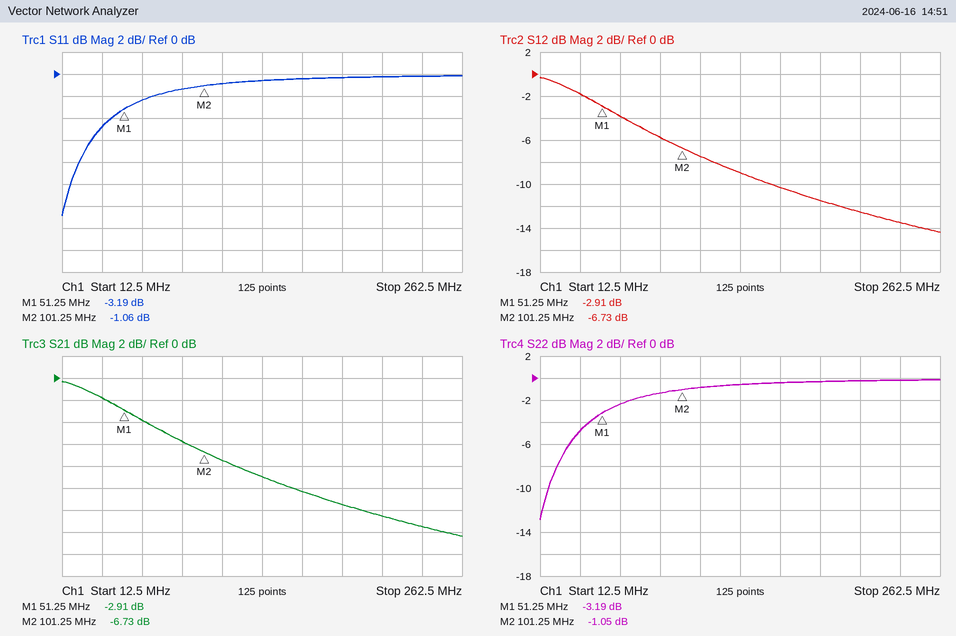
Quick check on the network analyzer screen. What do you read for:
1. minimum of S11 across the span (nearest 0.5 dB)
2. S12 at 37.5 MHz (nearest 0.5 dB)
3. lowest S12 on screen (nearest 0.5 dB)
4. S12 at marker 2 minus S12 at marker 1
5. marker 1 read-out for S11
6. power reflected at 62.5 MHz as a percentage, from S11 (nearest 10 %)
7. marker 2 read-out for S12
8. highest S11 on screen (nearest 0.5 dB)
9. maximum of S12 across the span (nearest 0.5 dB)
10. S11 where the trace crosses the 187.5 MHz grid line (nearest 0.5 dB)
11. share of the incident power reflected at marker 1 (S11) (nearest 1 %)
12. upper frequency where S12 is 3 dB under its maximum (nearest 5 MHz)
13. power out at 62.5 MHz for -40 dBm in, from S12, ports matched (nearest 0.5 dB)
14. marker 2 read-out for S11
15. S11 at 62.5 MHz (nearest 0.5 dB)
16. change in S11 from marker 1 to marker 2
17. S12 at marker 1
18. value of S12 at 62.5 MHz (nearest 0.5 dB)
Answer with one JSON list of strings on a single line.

["-13.0 dB", "-2.0 dB", "-14.5 dB", "-3.82 dB", "-3.19 dB", "60 %", "-6.73 dB", "0.0 dB", "-0.5 dB", "-0.5 dB", "48 %", "55 MHz", "-44.0 dBm", "-1.06 dB", "-2.5 dB", "2.13 dB", "-2.91 dB", "-4.0 dB"]
